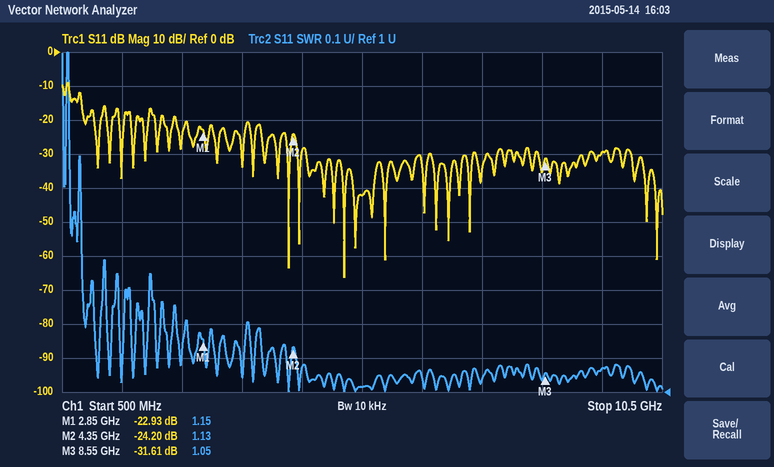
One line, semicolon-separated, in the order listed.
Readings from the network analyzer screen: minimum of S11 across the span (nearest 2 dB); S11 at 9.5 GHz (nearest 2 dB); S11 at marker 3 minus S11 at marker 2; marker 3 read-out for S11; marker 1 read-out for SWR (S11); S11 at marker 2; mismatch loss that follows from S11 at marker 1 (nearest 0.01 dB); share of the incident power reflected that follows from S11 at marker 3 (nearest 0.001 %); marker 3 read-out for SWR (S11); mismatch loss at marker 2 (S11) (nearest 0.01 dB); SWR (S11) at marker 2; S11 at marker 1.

-66 dB; -30 dB; -7.41 dB; -31.61 dB; 1.15; -24.20 dB; 0.02 dB; 0.069 %; 1.05; 0.02 dB; 1.13; -22.93 dB
